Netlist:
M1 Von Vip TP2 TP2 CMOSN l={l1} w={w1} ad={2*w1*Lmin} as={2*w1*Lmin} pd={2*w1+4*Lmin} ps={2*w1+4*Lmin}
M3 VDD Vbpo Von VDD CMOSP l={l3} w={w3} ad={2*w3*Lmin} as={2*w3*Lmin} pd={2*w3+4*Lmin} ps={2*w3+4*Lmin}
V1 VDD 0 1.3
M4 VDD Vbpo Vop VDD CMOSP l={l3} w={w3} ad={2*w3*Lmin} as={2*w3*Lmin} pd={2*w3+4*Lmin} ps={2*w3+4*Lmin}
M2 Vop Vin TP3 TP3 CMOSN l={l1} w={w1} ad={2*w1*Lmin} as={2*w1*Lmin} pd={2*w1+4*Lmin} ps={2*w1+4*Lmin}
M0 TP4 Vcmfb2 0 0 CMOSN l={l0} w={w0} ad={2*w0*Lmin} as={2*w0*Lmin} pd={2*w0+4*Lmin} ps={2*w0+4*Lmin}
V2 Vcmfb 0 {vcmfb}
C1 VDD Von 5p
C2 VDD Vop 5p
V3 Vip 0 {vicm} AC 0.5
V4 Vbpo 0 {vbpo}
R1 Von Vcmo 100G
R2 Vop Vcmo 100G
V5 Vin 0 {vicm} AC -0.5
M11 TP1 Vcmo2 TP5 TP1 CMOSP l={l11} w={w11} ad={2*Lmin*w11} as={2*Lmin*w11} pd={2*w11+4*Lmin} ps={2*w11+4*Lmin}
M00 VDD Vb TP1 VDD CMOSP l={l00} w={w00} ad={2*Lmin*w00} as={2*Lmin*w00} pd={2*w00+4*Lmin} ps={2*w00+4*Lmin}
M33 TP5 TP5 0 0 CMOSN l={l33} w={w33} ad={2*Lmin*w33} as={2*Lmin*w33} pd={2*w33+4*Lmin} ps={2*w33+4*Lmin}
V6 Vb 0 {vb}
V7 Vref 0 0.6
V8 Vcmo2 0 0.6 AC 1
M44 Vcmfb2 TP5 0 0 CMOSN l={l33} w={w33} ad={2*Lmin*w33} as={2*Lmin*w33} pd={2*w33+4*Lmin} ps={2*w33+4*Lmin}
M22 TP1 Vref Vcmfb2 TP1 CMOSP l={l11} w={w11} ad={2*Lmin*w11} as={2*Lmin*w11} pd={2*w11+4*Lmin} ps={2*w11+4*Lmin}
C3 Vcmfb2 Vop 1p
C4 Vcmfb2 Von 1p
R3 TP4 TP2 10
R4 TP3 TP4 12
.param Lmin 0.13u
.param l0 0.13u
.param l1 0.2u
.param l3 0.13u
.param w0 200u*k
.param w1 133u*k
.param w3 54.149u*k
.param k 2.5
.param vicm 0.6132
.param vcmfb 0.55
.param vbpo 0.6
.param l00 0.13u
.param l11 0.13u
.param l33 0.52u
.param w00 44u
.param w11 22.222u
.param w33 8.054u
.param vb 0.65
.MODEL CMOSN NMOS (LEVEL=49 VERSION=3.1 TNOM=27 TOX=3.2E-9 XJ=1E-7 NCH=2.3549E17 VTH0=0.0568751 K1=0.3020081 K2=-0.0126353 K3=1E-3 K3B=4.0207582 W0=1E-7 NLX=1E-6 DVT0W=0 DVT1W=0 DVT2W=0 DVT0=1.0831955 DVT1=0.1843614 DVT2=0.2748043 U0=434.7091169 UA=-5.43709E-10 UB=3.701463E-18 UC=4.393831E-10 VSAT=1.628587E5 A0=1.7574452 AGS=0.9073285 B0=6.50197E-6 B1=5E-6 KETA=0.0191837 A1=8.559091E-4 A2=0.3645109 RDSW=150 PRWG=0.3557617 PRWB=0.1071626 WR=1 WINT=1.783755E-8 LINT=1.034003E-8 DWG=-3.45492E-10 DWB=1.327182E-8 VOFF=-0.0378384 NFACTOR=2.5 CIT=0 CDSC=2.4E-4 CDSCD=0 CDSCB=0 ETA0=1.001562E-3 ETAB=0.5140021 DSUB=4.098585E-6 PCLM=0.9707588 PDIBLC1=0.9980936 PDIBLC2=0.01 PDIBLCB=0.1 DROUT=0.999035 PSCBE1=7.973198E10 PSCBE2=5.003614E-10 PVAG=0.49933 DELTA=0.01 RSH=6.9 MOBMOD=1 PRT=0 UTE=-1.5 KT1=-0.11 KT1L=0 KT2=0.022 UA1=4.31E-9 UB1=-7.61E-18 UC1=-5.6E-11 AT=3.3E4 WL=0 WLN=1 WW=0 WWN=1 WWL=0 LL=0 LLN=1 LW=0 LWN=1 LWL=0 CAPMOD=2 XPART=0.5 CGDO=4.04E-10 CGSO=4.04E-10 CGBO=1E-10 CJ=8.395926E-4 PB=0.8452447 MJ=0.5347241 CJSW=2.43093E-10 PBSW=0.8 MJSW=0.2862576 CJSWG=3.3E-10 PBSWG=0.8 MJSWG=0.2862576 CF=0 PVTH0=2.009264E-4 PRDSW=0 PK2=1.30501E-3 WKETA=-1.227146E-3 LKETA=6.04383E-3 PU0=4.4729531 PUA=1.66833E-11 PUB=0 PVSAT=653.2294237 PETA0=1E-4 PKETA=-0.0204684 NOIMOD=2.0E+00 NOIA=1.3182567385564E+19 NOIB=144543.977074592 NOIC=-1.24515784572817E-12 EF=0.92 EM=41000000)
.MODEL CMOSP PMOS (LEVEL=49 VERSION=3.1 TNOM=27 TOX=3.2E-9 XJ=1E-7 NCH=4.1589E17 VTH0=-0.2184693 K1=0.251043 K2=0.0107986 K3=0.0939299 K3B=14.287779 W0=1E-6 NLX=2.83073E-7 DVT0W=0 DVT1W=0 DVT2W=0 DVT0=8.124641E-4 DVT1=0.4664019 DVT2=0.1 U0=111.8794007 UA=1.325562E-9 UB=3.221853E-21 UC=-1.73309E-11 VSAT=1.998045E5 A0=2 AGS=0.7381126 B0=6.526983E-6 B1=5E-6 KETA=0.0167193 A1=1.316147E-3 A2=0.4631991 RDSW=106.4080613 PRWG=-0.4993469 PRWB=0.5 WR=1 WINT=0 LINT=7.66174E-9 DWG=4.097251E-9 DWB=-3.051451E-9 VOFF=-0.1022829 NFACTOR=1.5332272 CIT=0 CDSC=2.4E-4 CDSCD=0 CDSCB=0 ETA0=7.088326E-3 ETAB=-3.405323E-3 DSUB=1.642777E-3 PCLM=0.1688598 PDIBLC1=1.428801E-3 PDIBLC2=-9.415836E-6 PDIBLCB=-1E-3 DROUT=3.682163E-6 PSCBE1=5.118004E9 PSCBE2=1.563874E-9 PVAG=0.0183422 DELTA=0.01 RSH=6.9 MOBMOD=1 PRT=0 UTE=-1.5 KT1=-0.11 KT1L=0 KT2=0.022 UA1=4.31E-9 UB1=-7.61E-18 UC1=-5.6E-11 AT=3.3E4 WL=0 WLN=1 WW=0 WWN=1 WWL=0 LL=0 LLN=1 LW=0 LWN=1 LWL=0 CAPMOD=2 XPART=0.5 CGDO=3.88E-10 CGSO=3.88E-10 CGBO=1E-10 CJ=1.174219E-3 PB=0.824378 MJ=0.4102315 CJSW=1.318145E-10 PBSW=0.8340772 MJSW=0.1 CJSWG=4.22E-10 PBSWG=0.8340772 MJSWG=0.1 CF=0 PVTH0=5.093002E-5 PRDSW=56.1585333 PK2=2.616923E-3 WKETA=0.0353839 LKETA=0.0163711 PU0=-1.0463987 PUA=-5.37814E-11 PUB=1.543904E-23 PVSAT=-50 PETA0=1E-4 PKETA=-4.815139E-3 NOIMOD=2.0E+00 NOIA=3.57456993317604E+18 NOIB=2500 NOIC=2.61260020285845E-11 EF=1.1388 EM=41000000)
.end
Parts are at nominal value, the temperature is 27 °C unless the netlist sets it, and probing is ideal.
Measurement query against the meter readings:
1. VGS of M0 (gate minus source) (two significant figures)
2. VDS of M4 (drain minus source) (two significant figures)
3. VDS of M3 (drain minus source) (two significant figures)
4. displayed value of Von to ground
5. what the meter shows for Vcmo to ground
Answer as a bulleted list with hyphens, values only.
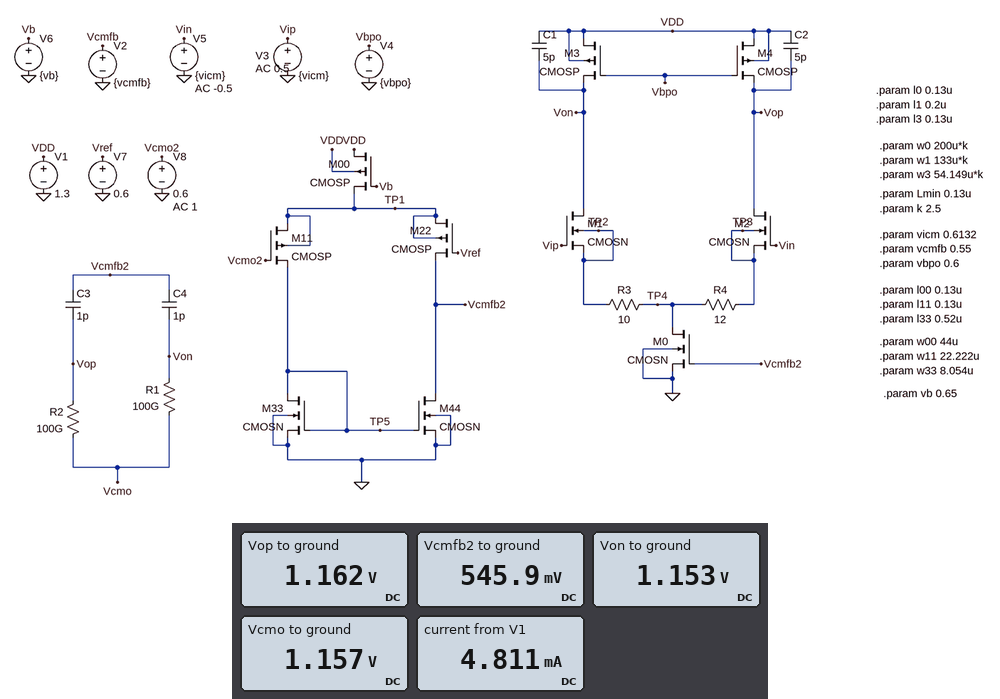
- 550 mV
- 140 mV
- 150 mV
- 1.153 V
- 1.157 V
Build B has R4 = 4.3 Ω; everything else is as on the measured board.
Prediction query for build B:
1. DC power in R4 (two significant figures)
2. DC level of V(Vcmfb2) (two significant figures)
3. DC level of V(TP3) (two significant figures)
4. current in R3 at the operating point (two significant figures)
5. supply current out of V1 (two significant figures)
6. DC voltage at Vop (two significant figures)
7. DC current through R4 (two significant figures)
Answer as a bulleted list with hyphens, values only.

- 23 µW
- 550 mV
- 180 mV
- 2.0 mA
- 4.9 mA
- 1.1 V
- 2.3 mA
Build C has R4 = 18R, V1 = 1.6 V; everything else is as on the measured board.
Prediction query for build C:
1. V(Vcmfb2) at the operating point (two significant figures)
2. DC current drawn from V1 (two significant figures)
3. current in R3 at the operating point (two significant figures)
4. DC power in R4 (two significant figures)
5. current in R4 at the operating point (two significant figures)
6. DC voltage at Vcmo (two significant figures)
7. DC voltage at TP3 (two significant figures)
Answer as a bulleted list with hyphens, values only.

- 920 mV
- 9.1 mA
- 3.9 mA
- 180 µW
- 3.1 mA
- 1.5 V
- 170 mV
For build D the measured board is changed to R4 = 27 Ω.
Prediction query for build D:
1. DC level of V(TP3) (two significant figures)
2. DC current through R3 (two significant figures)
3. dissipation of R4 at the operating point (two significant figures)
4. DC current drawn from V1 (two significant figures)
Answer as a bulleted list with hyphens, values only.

- 200 mV
- 2.4 mA
- 82 µW
- 4.7 mA
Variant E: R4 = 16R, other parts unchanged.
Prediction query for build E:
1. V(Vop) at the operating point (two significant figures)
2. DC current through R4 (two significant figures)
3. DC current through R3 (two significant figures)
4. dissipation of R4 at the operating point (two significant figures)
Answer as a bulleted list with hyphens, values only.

- 1.2 V
- 2.0 mA
- 2.3 mA
- 63 µW
